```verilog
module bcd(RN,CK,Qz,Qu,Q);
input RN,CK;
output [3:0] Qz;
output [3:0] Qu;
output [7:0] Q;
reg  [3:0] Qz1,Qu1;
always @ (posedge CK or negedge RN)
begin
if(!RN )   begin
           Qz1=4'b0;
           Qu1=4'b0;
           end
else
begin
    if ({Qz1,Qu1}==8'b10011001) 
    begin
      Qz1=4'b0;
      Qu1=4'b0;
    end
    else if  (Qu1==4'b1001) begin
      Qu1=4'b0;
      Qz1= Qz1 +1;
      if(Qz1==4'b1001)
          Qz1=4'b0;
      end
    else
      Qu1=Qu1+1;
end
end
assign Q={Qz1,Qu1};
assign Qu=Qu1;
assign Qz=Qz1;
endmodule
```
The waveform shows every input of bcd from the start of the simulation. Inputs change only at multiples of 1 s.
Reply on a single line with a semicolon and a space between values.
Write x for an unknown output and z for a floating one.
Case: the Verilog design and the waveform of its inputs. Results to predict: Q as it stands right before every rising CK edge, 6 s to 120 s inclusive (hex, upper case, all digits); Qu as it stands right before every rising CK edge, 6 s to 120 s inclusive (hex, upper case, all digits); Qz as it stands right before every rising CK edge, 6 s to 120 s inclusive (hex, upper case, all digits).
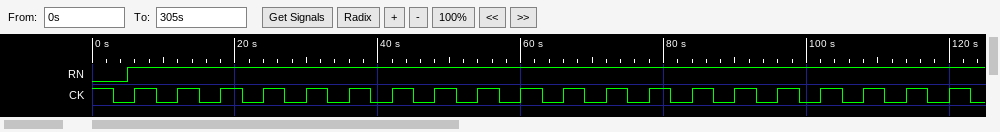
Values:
00, 01, 02, 03, 04, 05, 06, 07, 08, 09, 10, 11, 12, 13, 14, 15, 16, 17, 18, 19; 0, 1, 2, 3, 4, 5, 6, 7, 8, 9, 0, 1, 2, 3, 4, 5, 6, 7, 8, 9; 0, 0, 0, 0, 0, 0, 0, 0, 0, 0, 1, 1, 1, 1, 1, 1, 1, 1, 1, 1
